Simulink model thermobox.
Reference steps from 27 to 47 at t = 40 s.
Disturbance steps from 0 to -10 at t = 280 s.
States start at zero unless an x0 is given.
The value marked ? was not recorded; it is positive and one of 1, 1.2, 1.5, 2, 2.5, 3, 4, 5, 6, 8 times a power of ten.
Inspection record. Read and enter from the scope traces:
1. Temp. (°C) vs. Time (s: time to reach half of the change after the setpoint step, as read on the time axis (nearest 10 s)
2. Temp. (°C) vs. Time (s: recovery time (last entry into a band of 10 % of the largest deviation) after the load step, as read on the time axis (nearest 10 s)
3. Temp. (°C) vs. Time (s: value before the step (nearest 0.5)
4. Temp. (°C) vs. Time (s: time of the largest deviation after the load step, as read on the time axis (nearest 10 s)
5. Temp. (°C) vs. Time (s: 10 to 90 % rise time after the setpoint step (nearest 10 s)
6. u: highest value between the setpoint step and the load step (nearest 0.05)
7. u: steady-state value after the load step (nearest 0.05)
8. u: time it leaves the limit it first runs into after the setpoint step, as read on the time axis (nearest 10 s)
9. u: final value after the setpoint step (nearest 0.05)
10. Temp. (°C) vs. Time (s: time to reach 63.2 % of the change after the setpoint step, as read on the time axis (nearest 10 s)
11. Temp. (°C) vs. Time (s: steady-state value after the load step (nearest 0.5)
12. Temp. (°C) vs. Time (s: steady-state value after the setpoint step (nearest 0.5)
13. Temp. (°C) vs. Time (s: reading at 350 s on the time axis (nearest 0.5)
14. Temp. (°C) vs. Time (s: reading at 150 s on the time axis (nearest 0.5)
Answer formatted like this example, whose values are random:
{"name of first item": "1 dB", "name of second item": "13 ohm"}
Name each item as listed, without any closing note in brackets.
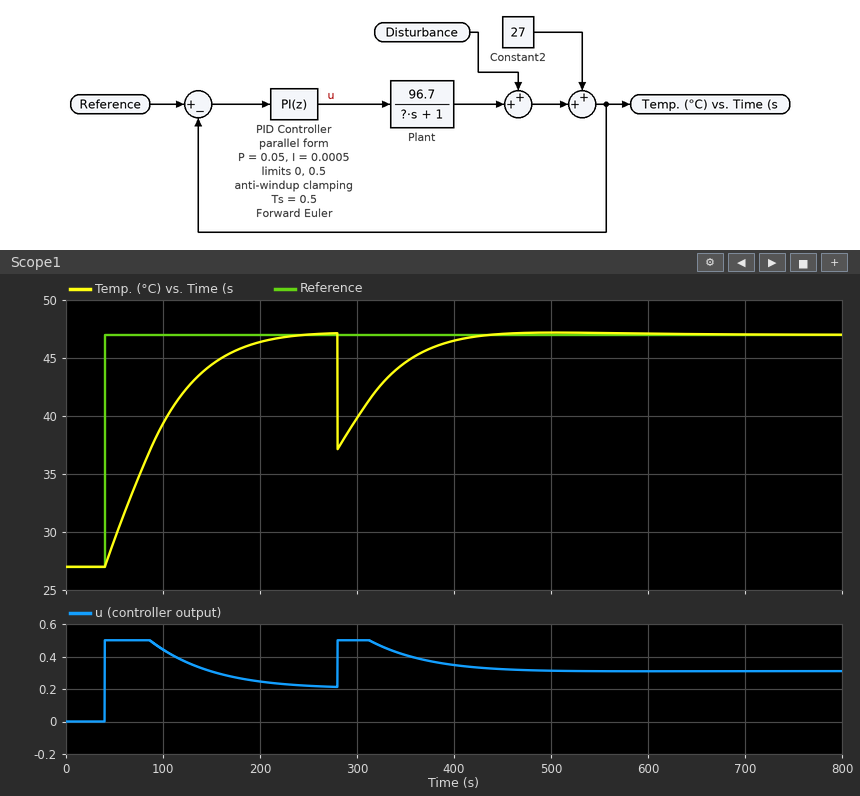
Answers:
{"Temp. (°C) vs. Time (s: time to reach half of the change after the setpoint step, as read on the time axis": "90 s", "Temp. (°C) vs. Time (s: recovery time (last entry into a band of 10 % of the largest deviation) after the load step, as read on the time axis": "380 s", "Temp. (°C) vs. Time (s: value before the step": "27.0", "Temp. (°C) vs. Time (s: time of the largest deviation after the load step, as read on the time axis": "280 s", "Temp. (°C) vs. Time (s: 10 to 90 % rise time after the setpoint step": "110 s", "u: highest value between the setpoint step and the load step": "0.50", "u: steady-state value after the load step": "0.30", "u: time it leaves the limit it first runs into after the setpoint step, as read on the time axis": "90 s", "u: final value after the setpoint step": "0.20", "Temp. (°C) vs. Time (s: time to reach 63.2 % of the change after the setpoint step, as read on the time axis": "100 s", "Temp. (°C) vs. Time (s: steady-state value after the load step": "47.0", "Temp. (°C) vs. Time (s: steady-state value after the setpoint step": "47.0", "Temp. (°C) vs. Time (s: reading at 350 s on the time axis": "44.5", "Temp. (°C) vs. Time (s: reading at 150 s on the time axis": "44.5"}
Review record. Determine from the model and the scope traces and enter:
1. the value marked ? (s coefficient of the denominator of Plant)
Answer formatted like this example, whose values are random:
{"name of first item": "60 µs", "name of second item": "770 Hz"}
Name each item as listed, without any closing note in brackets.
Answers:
{"the value marked ?": "200"}
